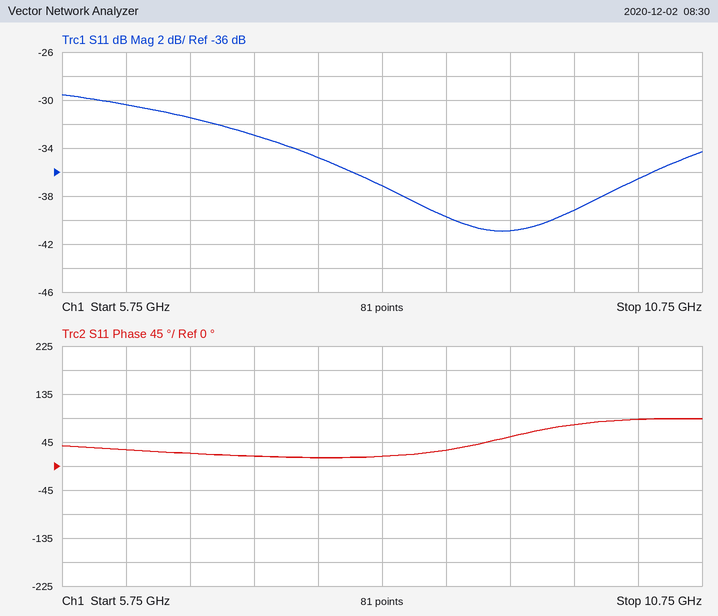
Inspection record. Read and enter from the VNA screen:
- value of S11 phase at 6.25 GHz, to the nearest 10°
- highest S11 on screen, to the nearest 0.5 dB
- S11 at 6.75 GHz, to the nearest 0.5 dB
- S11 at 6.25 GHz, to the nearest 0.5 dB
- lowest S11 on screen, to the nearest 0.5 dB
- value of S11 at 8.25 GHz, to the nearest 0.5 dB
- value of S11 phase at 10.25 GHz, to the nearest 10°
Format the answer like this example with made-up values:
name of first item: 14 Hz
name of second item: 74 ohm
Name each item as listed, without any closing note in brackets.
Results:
value of S11 phase at 6.25 GHz, to the nearest 10°: 30°
highest S11 on screen, to the nearest 0.5 dB: -29.5 dB
S11 at 6.75 GHz, to the nearest 0.5 dB: -31.5 dB
S11 at 6.25 GHz, to the nearest 0.5 dB: -30.5 dB
lowest S11 on screen, to the nearest 0.5 dB: -41.0 dB
value of S11 at 8.25 GHz, to the nearest 0.5 dB: -37.0 dB
value of S11 phase at 10.25 GHz, to the nearest 10°: 90°
